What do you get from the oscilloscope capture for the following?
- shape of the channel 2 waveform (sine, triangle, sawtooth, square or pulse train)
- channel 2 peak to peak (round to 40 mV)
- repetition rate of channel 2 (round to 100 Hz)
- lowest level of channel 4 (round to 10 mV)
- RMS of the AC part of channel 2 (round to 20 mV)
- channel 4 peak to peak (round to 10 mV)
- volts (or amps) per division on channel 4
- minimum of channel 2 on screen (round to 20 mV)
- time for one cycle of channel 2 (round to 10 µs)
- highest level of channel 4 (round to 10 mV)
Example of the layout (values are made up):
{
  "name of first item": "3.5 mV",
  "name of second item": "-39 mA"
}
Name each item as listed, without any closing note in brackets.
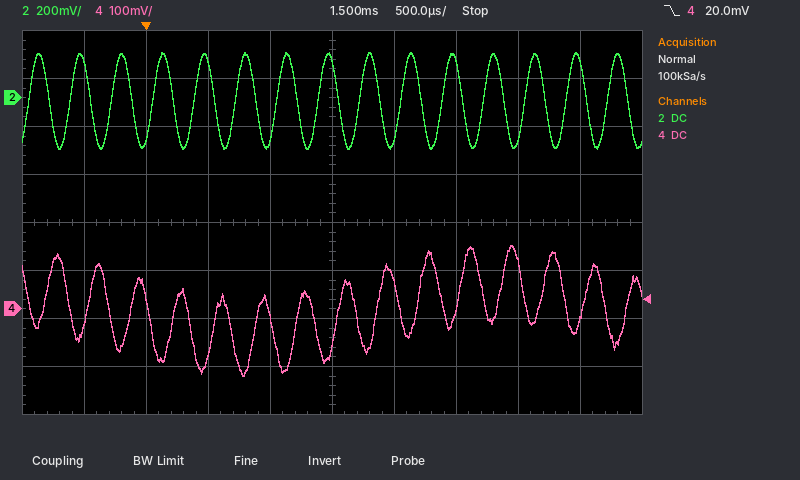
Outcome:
{
  "shape of the channel 2 waveform": "sine",
  "channel 2 peak to peak": "400 mV",
  "repetition rate of channel 2": "3.0 kHz",
  "lowest level of channel 4": "-140 mV",
  "RMS of the AC part of channel 2": "140 mV",
  "channel 4 peak to peak": "270 mV",
  "volts (or amps) per division on channel 4": "100 mV",
  "minimum of channel 2 on screen": "-220 mV",
  "time for one cycle of channel 2": "330 µs",
  "highest level of channel 4": "130 mV"
}
